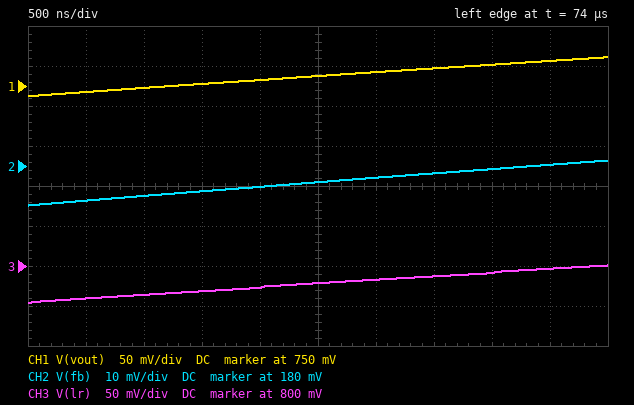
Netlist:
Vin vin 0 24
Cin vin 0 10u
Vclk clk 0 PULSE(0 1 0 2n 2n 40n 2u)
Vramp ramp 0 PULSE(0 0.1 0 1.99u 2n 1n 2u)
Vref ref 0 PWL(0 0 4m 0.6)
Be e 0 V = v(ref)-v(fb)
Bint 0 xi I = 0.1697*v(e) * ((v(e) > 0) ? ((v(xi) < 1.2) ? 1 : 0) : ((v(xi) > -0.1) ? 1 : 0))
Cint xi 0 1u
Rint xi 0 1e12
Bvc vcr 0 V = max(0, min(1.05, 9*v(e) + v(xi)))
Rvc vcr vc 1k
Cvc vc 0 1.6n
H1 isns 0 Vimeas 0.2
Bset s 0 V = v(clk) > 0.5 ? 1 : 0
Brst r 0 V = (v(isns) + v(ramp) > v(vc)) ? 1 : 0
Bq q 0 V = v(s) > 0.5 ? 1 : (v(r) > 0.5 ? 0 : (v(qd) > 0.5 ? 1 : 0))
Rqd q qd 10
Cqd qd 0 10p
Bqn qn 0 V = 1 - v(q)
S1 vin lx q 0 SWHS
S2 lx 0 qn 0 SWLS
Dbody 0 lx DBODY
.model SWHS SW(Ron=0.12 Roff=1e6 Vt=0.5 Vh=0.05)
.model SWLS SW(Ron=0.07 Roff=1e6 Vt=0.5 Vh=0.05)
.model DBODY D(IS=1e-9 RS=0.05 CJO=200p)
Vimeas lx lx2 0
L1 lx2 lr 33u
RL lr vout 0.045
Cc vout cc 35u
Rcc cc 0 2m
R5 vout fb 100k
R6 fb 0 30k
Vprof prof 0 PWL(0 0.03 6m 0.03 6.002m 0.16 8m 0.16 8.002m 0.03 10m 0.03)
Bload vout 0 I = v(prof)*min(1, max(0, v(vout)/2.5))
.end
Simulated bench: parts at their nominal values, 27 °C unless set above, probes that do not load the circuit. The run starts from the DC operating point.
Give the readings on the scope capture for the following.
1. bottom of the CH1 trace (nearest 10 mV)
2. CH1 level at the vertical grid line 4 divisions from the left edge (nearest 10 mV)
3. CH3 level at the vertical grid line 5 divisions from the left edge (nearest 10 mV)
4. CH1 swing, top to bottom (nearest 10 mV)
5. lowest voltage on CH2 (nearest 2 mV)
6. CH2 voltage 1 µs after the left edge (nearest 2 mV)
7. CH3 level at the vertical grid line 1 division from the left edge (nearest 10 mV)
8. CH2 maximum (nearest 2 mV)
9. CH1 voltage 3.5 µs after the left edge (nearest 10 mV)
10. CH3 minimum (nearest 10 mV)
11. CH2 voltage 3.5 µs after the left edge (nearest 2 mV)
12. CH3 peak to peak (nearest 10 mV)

740 mV
760 mV
780 mV
50 mV
170 mV
172 mV
760 mV
182 mV
770 mV
750 mV
178 mV
50 mV
